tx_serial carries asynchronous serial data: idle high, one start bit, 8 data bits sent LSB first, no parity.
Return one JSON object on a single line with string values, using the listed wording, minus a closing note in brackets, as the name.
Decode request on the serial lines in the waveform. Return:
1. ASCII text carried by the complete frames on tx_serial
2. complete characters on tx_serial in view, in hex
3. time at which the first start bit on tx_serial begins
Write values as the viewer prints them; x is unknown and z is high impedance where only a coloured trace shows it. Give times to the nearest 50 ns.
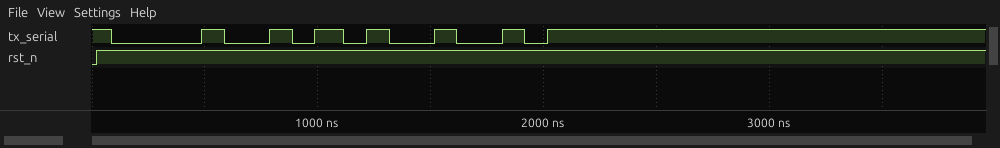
{"ASCII text carried by the complete frames on tx_serial": "\"HI\"", "complete characters on tx_serial in view, in hex": "48, 49", "time at which the first start bit on tx_serial begins": "100 ns"}
